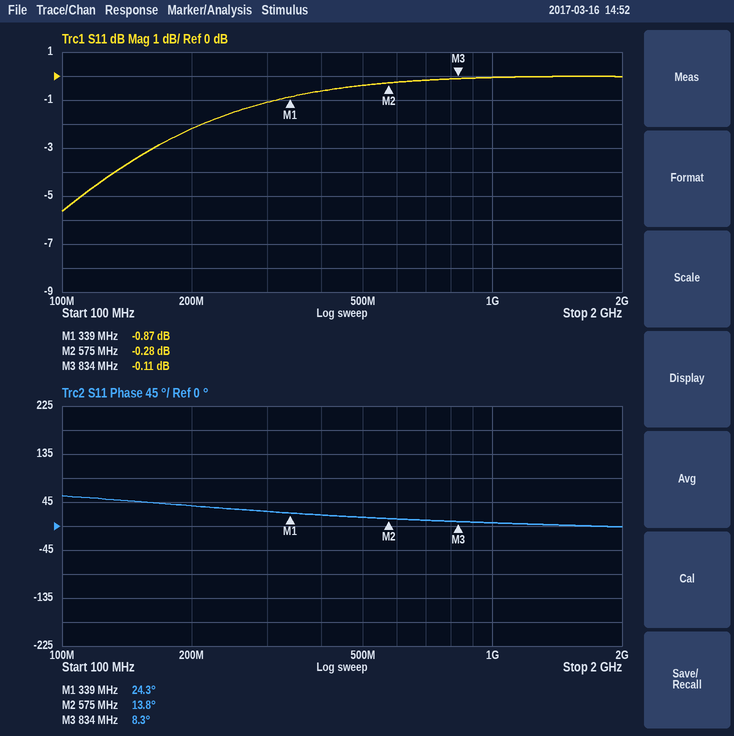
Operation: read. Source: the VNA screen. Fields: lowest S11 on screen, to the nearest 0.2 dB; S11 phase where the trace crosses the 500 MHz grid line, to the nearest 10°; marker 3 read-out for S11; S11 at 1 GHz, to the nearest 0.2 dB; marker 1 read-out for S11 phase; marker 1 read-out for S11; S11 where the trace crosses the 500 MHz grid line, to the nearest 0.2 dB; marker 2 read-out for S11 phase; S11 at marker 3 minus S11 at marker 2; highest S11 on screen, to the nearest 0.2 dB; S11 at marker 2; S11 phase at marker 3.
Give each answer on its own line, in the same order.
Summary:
-5.6 dB
20°
-0.11 dB
0.0 dB
24.3°
-0.87 dB
-0.4 dB
13.8°
0.17 dB
0.0 dB
-0.28 dB
8.3°
